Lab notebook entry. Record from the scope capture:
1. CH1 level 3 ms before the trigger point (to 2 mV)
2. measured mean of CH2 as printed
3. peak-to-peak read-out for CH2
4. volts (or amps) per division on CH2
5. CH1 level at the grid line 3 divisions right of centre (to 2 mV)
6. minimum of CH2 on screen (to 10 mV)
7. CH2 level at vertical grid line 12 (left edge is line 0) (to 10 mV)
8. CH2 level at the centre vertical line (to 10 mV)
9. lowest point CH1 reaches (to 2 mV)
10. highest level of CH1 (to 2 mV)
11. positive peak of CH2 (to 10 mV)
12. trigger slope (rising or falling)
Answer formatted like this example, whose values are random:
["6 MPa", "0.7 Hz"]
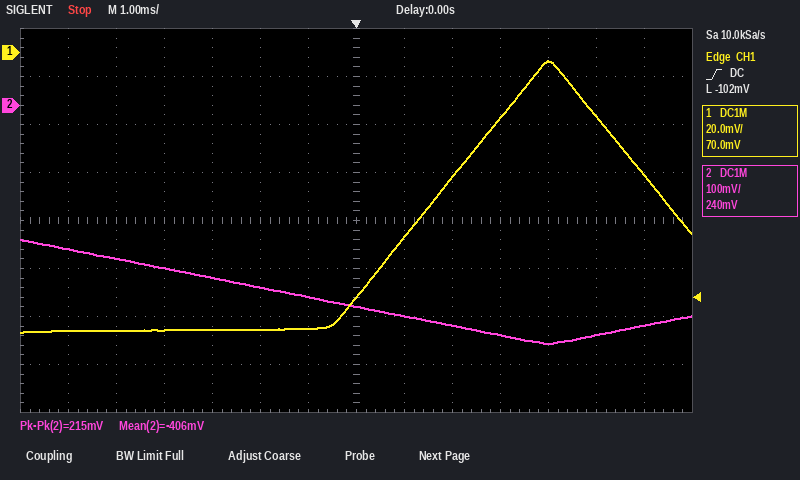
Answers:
["-116 mV", "-406 mV", "215 mV", "100 mV", "-28 mV", "-500 mV", "-480 mV", "-420 mV", "-116 mV", "-4 mV", "-280 mV", "rising"]
